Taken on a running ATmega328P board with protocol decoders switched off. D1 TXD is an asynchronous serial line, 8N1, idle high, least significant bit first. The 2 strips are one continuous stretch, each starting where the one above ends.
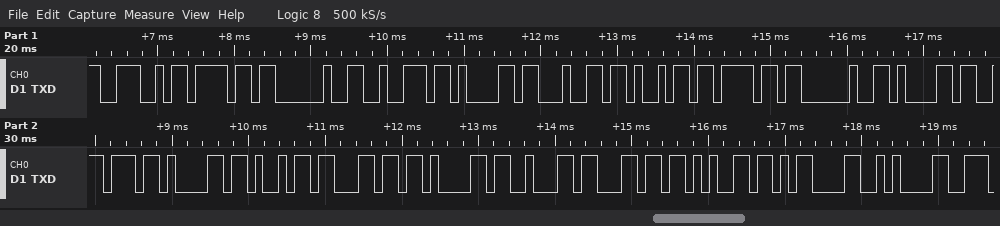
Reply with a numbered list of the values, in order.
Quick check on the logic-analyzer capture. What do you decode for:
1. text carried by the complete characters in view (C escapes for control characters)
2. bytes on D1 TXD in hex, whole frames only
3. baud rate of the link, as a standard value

1. "No radio available\r\n"
2. 4E 6F 20 72 61 64 69 6F 20 61 76 61 69 6C 61 62 6C 65 0D 0A
3. 9600 baud
